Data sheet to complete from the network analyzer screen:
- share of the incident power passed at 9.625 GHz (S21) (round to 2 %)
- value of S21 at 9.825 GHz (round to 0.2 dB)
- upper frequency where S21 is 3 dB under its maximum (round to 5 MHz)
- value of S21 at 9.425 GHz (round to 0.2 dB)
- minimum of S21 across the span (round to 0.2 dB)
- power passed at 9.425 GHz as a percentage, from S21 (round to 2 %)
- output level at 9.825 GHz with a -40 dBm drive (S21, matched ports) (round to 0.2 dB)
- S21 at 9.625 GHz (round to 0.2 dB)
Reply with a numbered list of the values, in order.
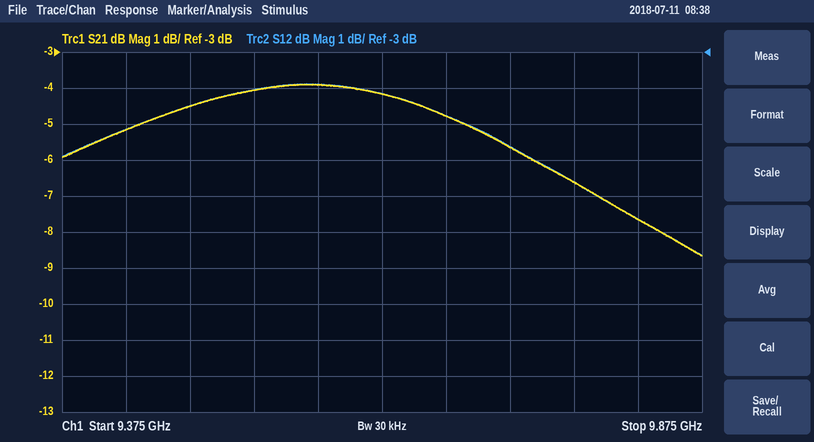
1. 38 %
2. -7.6 dB
3. 9.790 GHz
4. -5.2 dB
5. -8.6 dB
6. 30 %
7. -47.6 dBm
8. -4.2 dB
